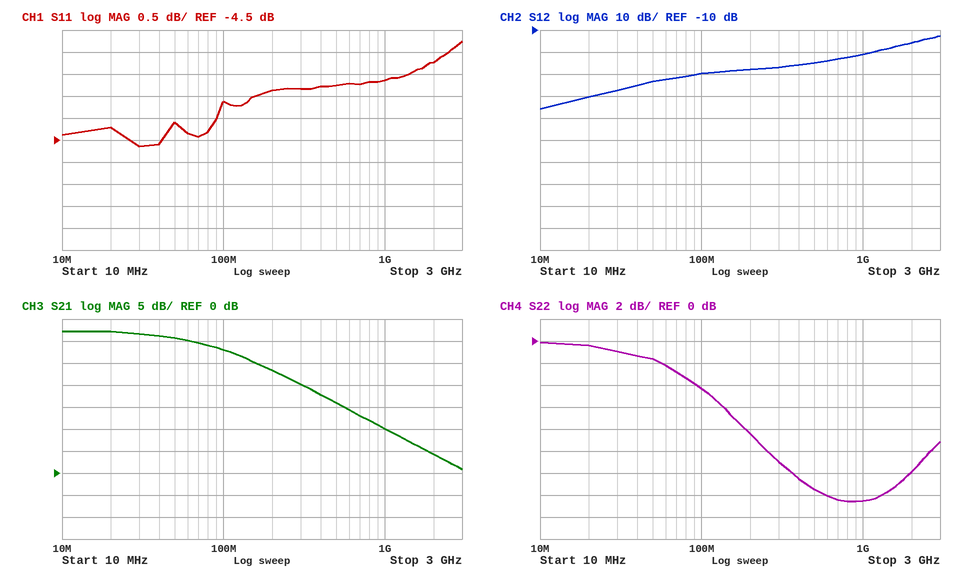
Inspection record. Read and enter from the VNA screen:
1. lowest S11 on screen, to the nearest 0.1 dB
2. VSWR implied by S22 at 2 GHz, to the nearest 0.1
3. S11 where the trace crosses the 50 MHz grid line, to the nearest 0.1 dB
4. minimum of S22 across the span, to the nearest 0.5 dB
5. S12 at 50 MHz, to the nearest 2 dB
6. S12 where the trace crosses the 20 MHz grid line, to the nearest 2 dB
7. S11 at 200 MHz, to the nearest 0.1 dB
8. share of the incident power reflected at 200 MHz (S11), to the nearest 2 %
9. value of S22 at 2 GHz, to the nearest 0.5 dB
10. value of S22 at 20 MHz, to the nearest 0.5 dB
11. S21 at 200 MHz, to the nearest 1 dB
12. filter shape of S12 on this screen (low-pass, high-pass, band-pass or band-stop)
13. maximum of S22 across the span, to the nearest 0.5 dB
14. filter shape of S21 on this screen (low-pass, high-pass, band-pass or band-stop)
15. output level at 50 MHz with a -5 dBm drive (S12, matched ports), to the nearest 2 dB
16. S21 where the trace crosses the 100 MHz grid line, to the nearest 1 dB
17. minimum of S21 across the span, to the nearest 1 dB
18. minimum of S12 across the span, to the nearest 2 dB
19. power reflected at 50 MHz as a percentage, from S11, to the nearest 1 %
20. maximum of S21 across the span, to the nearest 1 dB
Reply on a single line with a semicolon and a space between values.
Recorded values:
-4.6 dB; 1.7; -4.1 dB; -14.5 dB; -34 dB; -40 dB; -3.4 dB; 46 %; -12.0 dB; -0.5 dB; 23 dB; high-pass; 0.0 dB; low-pass; -38 dBm; 28 dB; 1 dB; -46 dB; 39 %; 32 dB
